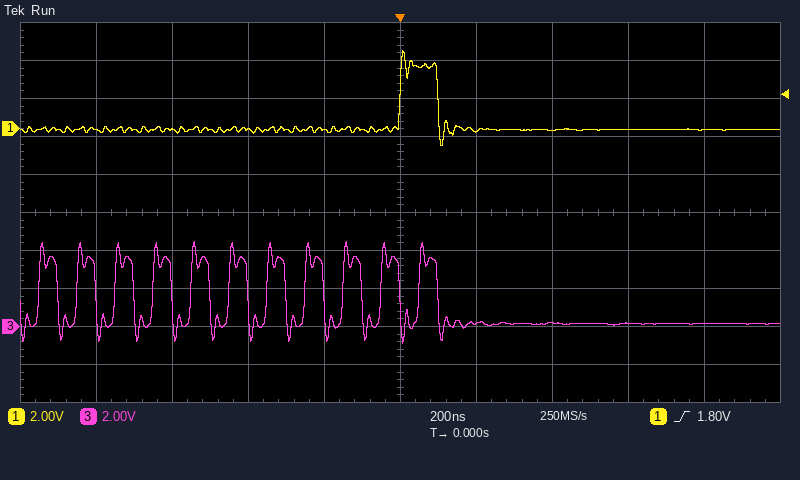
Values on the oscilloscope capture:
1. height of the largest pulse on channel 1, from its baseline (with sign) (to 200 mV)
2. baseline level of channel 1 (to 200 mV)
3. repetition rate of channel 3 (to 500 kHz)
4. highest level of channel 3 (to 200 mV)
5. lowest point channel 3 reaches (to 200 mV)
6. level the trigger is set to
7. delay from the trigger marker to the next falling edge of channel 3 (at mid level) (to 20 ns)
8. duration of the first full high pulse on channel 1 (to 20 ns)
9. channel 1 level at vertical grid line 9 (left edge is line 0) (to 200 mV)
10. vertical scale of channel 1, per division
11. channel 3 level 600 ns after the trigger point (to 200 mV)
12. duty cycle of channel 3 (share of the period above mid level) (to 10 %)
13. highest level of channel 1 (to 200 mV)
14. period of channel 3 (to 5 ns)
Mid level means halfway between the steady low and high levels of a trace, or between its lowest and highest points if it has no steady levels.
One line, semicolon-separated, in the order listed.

+4.2 V; 0.0 V; 10.0 MHz; 4.4 V; -800 mV; 1.80 V; 100 ns; 100 ns; 0.0 V; 2 V; 200 mV; 50 %; 4.2 V; 100 ns
